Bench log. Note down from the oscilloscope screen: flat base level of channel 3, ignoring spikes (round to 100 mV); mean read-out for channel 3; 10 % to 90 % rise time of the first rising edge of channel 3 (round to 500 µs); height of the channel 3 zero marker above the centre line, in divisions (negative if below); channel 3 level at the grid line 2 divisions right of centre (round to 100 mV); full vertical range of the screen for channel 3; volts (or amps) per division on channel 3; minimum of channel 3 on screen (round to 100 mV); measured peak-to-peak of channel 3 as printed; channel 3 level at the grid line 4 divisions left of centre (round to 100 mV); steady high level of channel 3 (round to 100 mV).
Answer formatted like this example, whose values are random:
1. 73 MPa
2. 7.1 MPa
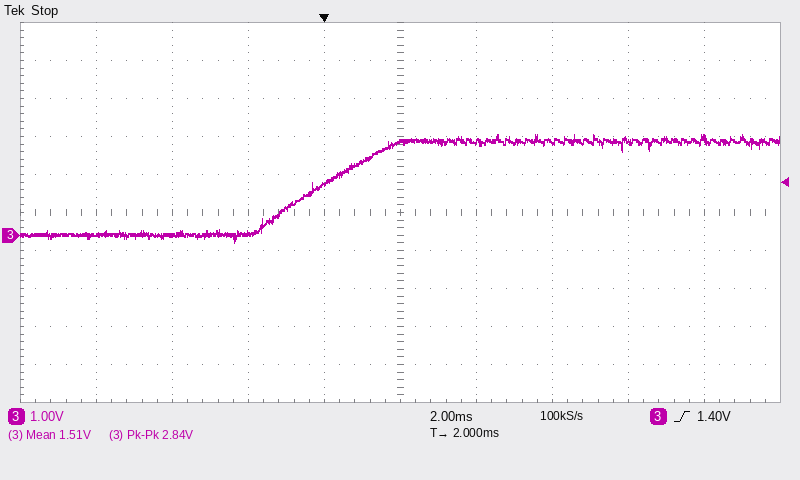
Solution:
1. 0.0 V
2. 1.51 V
3. 3.0 ms
4. -0.6 div
5. 2.5 V
6. 10 V
7. 1 V
8. -200 mV
9. 2.84 V
10. 0.0 V
11. 2.5 V
